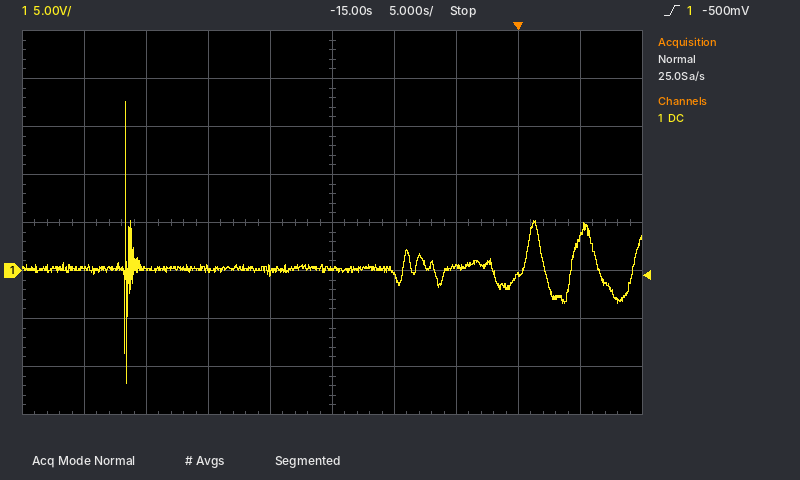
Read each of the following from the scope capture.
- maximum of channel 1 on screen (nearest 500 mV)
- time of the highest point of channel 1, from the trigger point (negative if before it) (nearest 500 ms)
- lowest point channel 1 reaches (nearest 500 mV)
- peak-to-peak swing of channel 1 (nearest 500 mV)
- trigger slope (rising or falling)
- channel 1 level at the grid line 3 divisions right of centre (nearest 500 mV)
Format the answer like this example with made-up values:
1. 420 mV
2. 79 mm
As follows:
1. 17.5 V
2. -31.5 s
3. -12.0 V
4. 29.5 V
5. rising
6. -500 mV
